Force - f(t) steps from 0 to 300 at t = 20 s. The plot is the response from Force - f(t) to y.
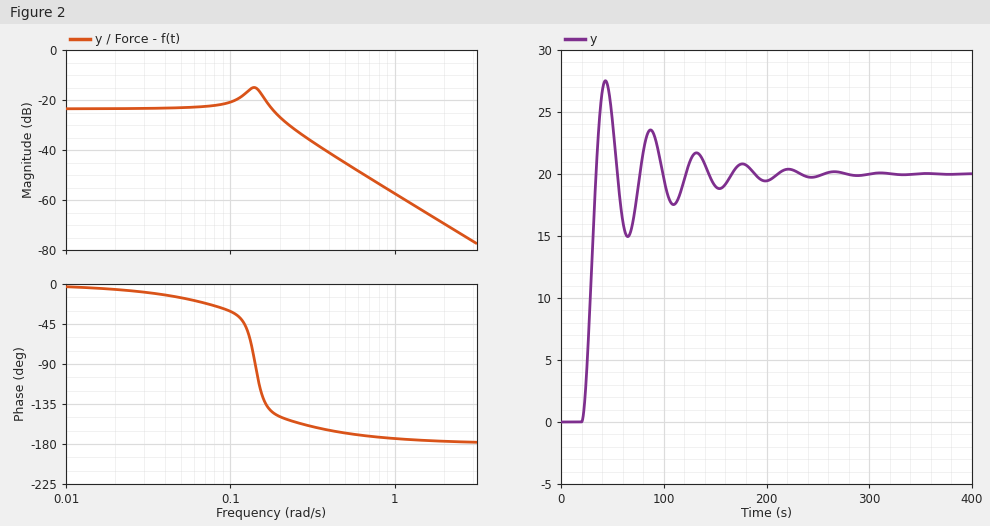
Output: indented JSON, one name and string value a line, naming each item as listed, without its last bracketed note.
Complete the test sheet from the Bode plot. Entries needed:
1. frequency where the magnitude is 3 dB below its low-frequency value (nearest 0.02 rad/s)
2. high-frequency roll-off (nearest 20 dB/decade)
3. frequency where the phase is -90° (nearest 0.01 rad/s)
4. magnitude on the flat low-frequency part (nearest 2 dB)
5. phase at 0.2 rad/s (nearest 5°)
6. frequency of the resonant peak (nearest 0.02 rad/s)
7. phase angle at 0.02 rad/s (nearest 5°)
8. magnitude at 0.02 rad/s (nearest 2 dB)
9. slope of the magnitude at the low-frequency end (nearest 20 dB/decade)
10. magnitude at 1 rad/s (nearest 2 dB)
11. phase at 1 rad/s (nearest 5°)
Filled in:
{
  "frequency where the magnitude is 3 dB below its low-frequency value": "0.20 rad/s",
  "high-frequency roll-off": "-40 dB/decade",
  "frequency where the phase is -90°": "0.14 rad/s",
  "magnitude on the flat low-frequency part": "-24 dB",
  "phase at 0.2 rad/s": "-150°",
  "frequency of the resonant peak": "0.14 rad/s",
  "phase angle at 0.02 rad/s": "-5°",
  "magnitude at 0.02 rad/s": "-24 dB",
  "slope of the magnitude at the low-frequency end": "0 dB/decade",
  "magnitude at 1 rad/s": "-58 dB",
  "phase at 1 rad/s": "-175°"
}
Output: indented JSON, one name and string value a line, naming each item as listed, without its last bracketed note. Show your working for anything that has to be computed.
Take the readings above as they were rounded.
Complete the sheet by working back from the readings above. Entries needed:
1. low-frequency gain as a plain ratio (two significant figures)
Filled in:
{
  "low-frequency gain as a plain ratio": "10^(-24 / 20) = 0.063"
}
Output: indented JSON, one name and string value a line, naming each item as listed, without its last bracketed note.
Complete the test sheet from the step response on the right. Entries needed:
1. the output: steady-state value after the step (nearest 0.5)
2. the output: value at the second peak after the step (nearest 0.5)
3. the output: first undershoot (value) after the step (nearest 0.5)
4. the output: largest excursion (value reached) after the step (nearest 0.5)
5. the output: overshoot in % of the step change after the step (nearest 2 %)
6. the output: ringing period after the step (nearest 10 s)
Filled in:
{
  "the output: steady-state value after the step": "20.0",
  "the output: value at the second peak after the step": "23.5",
  "the output: first undershoot (value) after the step": "15.0",
  "the output: largest excursion (value reached) after the step": "27.5",
  "the output: overshoot in % of the step change after the step": "38 %",
  "the output: ringing period after the step": "40 s"
}
